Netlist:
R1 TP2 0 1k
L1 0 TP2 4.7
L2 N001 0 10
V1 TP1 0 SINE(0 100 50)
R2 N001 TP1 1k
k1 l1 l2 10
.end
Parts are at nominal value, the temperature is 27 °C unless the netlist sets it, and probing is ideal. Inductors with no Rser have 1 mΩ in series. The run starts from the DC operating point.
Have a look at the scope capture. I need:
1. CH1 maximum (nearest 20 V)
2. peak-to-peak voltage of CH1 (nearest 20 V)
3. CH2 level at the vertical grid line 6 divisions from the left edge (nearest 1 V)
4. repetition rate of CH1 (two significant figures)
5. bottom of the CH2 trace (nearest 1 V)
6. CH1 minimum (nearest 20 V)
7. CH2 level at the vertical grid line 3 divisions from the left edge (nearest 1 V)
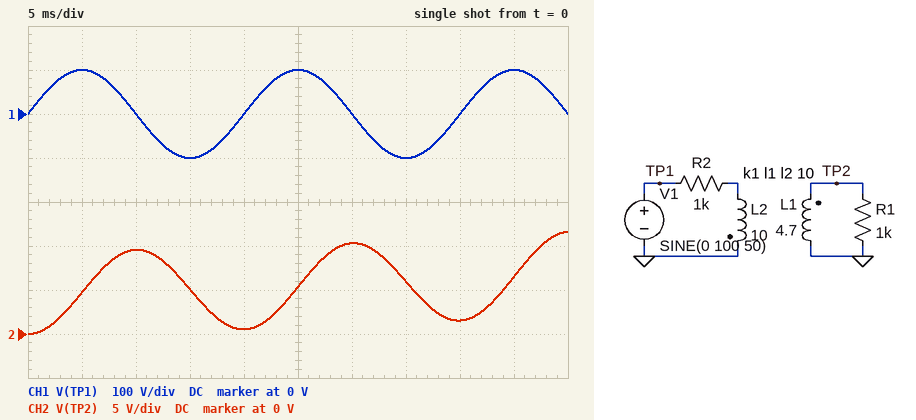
100 V
200 V
10 V
50 Hz
0 V
-100 V
5 V
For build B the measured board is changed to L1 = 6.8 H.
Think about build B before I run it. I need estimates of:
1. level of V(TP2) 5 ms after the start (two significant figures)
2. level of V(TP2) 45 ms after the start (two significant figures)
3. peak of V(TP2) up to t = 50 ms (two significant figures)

3.9 V
5.0 V
9.1 V
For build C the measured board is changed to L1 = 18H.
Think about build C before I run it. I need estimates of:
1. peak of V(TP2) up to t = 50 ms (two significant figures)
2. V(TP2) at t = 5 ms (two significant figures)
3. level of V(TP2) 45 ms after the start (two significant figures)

5.2 V
2.4 V
2.7 V
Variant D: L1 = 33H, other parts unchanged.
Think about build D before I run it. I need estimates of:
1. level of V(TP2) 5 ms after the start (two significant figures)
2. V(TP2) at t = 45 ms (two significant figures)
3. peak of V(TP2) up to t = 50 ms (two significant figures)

1.8 V
1.9 V
3.7 V
